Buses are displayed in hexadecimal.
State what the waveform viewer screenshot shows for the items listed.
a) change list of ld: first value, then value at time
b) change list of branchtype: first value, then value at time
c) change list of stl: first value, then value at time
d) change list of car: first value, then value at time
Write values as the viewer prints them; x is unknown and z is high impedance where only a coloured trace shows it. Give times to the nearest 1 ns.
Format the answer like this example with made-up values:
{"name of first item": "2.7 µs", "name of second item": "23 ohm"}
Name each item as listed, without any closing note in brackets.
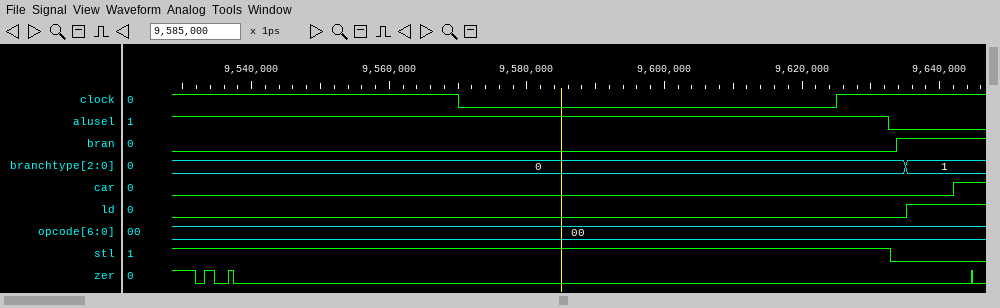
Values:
{"change list of ld: first value, then value at time": "0, 1 at 9635 ns", "change list of branchtype: first value, then value at time": "0, 1 at 9635 ns", "change list of stl: first value, then value at time": "1, 0 at 9633 ns", "change list of car: first value, then value at time": "0, 1 at 9642 ns"}
